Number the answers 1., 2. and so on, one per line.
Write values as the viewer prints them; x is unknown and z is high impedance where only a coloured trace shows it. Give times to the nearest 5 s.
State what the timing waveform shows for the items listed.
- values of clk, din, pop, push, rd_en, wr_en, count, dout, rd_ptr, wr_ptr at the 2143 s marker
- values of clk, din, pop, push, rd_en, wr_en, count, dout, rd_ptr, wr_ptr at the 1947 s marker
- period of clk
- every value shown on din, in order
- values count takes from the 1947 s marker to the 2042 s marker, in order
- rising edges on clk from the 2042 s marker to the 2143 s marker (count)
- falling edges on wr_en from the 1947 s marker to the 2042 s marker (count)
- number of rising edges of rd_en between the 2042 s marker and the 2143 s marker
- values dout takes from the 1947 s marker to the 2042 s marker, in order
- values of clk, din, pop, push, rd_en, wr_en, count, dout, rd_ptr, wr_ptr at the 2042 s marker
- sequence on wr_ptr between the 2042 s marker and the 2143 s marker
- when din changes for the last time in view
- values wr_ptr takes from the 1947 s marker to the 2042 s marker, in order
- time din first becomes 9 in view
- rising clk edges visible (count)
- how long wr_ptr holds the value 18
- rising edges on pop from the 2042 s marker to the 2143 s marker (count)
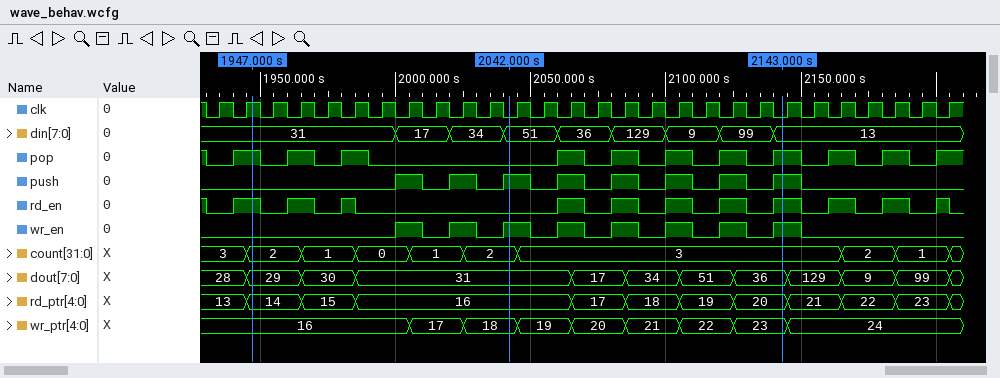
1. clk=0, din=13, pop=1, push=1, rd_en=1, wr_en=1, count=3, dout=36, rd_ptr=20, wr_ptr=23
2. clk=1, din=31, pop=1, push=0, rd_en=1, wr_en=0, count=2, dout=29, rd_ptr=14, wr_ptr=16
3. 10 s
4. 31, 17, 34, 51, 36, 129, 9, 99, 13
5. 2, 1, 0, 1, 2
6. 10
7. 2
8. 5
9. 29, 30, 31
10. clk=0, din=51, pop=0, push=1, rd_en=0, wr_en=1, count=2, dout=31, rd_ptr=16, wr_ptr=18
11. 18, 19, 20, 21, 22, 23
12. 2140 s
13. 16, 17, 18
14. 2100 s
15. 28
16. 20 s
17. 5
